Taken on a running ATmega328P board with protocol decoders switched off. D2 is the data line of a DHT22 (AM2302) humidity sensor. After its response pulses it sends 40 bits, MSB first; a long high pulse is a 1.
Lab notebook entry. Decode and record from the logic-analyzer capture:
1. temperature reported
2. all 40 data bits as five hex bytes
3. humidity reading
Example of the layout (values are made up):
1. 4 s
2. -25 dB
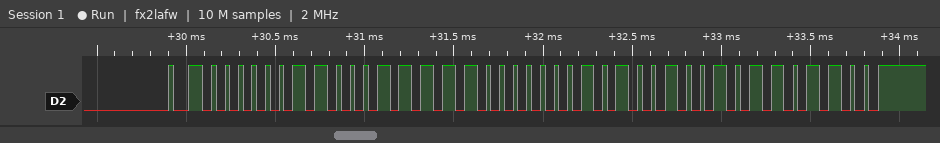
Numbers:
1. 32.9 °C
2. 03 1F 01 49 6C
3. 79.9 %
